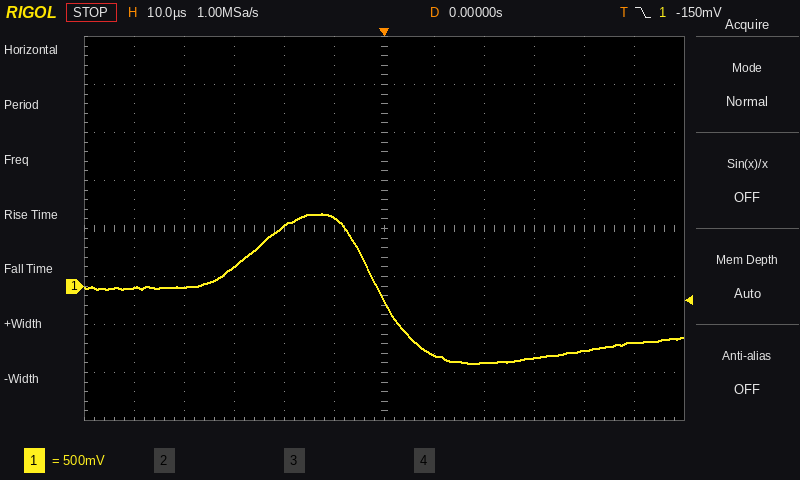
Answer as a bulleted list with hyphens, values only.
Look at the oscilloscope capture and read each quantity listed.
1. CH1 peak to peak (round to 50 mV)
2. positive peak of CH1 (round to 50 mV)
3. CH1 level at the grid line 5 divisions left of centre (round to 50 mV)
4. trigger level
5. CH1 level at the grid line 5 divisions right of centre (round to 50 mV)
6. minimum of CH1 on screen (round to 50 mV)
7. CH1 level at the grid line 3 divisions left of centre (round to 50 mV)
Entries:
- 1.55 V
- 750 mV
- 0 mV
- -150 mV
- -600 mV
- -800 mV
- 200 mV
